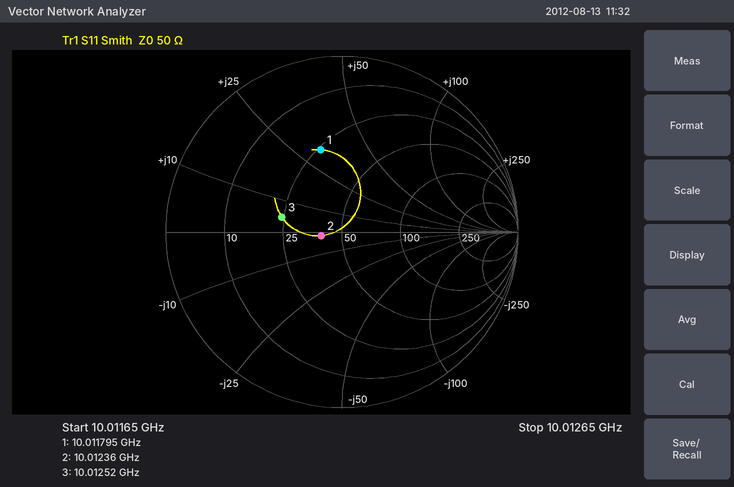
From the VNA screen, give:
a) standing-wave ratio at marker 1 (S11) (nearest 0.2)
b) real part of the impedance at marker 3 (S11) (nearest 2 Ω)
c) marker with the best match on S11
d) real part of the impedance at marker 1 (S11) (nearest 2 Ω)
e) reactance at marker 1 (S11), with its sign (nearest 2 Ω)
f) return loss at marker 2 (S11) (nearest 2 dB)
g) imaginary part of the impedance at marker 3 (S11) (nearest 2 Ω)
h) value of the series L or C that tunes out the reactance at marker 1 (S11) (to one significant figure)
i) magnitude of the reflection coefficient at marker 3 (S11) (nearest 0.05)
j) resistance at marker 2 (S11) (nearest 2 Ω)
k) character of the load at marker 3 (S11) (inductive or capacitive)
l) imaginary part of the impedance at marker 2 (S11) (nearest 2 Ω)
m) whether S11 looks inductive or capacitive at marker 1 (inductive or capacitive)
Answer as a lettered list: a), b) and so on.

a) 2.8
b) 24 Ω
c) marker 2
d) 26 Ω
e) +32 Ω
f) 18 dB
g) +4 Ω
h) 500 fF
i) 0.35
j) 40 Ω
k) inductive
l) -2 Ω
m) inductive
